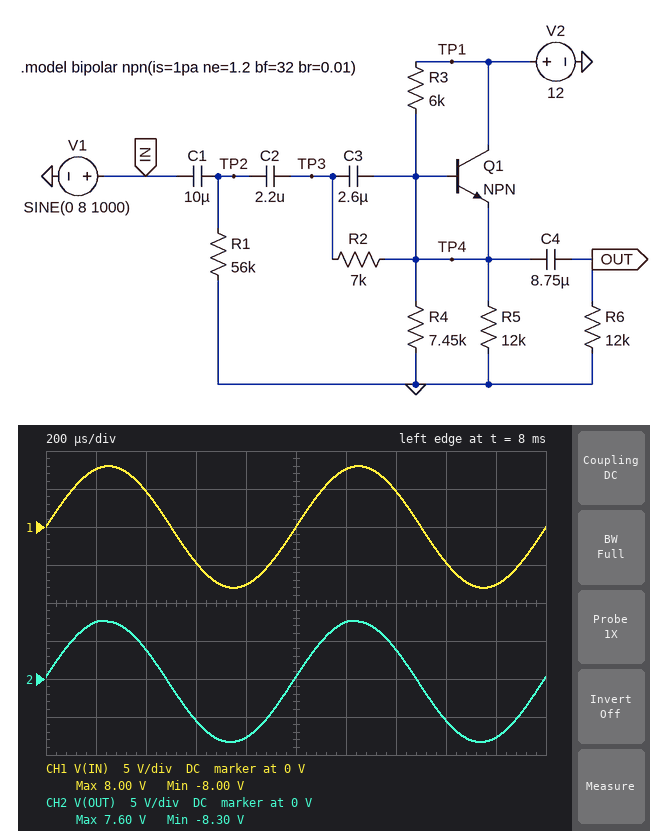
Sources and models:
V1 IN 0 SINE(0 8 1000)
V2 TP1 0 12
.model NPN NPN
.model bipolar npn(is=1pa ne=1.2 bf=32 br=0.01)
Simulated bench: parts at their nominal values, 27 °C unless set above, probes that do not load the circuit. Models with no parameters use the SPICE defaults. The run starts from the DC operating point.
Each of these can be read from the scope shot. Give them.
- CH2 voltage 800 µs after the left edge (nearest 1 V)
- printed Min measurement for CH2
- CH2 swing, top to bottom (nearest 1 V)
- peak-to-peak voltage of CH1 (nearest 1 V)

-8 V
-8.30 V
16 V
16 V
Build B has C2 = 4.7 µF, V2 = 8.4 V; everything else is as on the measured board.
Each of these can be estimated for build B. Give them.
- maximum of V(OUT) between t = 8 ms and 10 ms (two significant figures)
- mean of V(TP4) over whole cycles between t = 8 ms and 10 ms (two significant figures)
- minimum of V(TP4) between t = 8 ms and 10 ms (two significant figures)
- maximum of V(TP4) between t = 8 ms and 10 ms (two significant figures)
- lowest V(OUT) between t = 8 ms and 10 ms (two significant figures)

5.8 V
1.5 V
-6.4 V
9.2 V
-9.9 V
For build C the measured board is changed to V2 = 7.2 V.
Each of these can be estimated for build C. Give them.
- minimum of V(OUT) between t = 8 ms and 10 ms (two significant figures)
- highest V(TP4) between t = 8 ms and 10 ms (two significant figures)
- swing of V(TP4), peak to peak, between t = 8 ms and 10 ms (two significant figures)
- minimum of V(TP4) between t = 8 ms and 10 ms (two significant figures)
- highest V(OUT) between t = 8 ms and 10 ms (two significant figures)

-10 V
8.0 V
15 V
-7.4 V
5.1 V
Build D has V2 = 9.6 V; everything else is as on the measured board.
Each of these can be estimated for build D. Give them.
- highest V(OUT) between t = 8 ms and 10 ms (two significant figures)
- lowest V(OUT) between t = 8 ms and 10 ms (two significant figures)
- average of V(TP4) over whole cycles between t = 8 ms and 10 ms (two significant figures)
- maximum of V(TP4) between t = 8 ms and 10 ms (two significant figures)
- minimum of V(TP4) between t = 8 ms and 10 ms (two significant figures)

6.4 V
-9.3 V
2.7 V
10 V
-5.2 V
